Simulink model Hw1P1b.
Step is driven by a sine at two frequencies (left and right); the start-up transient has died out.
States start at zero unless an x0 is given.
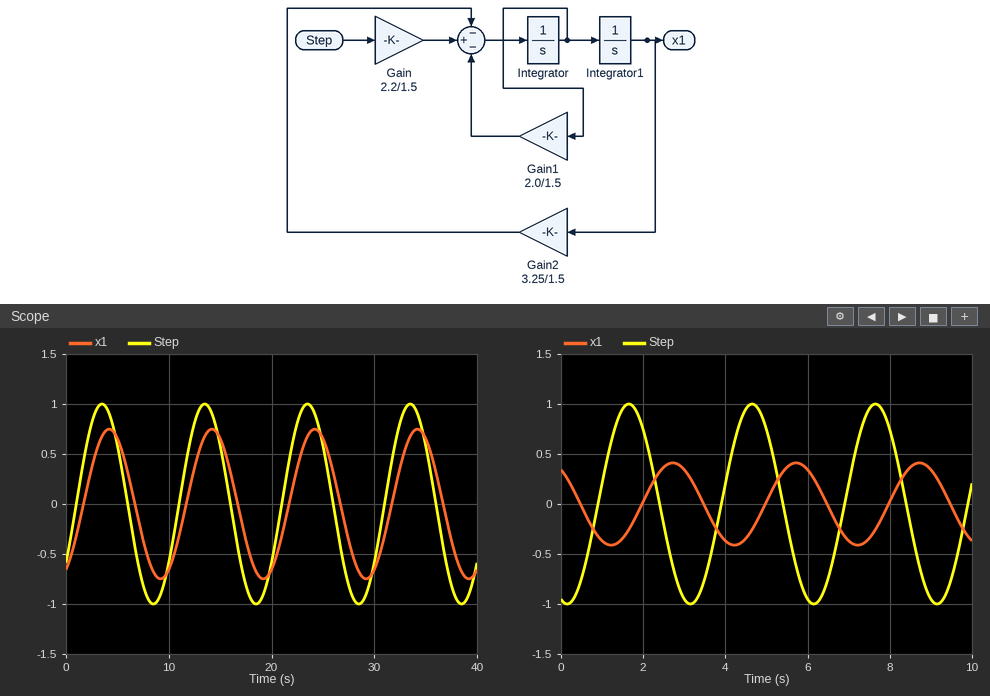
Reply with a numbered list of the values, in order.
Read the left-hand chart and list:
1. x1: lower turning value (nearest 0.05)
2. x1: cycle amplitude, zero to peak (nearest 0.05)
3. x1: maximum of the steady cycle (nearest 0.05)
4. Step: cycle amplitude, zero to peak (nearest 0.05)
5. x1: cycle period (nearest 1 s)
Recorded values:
1. -0.75
2. 0.75
3. 0.75
4. 1.00
5. 10 s
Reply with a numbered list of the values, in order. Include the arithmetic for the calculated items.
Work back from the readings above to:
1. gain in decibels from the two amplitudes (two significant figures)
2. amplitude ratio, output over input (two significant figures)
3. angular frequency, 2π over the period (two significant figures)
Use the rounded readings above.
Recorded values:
1. 20 log10(0.75 / 1) = -2.5 dB
2. 0.75 / 1 = 0.75
3. 2π / 10 = 0.63 rad/s
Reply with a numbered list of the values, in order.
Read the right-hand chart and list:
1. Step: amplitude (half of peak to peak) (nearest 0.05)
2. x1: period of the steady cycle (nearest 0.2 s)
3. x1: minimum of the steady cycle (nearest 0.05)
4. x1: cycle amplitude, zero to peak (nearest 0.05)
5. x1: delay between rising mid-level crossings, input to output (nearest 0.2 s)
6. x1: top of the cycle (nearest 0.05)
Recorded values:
1. 1.00
2. 3.0 s
3. -0.40
4. 0.40
5. 1.0 s
6. 0.40
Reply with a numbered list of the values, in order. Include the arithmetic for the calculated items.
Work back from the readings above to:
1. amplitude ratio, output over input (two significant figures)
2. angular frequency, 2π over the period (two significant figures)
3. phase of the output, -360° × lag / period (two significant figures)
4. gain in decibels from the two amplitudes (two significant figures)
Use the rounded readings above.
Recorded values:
1. 0.4 / 1 = 0.40
2. 2π / 3 = 2.1 rad/s
3. -360 × 1 / 3 = -120°
4. 20 log10(0.4 / 1) = -8.0 dB
